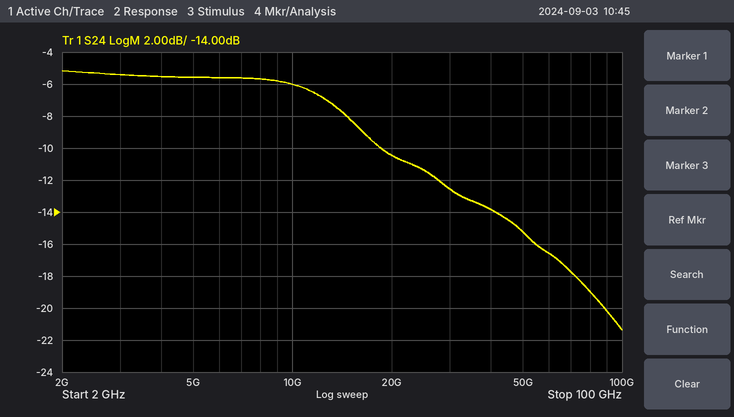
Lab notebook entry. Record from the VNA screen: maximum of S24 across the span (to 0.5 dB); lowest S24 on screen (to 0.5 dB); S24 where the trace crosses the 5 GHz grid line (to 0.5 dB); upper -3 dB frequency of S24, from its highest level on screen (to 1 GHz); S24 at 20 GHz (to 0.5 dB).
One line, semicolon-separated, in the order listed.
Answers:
-5.0 dB; -21.5 dB; -5.5 dB; 15 GHz; -10.5 dB
